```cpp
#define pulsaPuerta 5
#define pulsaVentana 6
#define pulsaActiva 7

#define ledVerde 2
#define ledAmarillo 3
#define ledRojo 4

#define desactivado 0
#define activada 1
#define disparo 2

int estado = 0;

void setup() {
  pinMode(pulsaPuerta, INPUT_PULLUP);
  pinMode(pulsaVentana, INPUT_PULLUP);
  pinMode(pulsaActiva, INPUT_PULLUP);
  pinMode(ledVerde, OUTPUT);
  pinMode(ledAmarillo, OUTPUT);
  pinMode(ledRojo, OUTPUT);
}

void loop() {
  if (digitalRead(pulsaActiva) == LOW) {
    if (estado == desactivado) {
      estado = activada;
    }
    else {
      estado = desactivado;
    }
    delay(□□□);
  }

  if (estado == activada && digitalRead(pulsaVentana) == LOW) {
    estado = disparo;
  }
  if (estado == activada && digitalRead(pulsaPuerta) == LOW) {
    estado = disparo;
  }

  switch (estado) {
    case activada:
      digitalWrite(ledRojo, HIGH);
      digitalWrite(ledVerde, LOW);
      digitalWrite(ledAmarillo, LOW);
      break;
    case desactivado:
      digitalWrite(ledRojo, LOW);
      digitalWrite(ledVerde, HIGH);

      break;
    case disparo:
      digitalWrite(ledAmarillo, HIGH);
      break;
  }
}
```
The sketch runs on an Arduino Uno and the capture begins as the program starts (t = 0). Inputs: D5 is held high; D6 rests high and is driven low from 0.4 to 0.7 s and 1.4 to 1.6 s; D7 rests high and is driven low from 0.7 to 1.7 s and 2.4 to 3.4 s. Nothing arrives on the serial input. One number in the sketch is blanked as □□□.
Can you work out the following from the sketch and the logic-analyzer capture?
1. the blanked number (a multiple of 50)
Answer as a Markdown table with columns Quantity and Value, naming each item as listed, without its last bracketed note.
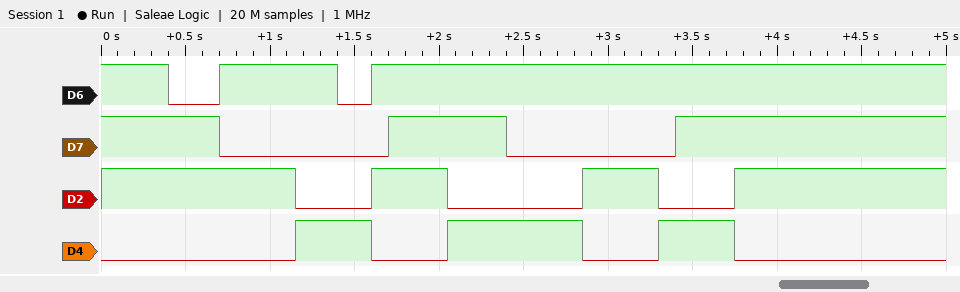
| Quantity | Value |
|---|---|
| the blanked number | 450 |
